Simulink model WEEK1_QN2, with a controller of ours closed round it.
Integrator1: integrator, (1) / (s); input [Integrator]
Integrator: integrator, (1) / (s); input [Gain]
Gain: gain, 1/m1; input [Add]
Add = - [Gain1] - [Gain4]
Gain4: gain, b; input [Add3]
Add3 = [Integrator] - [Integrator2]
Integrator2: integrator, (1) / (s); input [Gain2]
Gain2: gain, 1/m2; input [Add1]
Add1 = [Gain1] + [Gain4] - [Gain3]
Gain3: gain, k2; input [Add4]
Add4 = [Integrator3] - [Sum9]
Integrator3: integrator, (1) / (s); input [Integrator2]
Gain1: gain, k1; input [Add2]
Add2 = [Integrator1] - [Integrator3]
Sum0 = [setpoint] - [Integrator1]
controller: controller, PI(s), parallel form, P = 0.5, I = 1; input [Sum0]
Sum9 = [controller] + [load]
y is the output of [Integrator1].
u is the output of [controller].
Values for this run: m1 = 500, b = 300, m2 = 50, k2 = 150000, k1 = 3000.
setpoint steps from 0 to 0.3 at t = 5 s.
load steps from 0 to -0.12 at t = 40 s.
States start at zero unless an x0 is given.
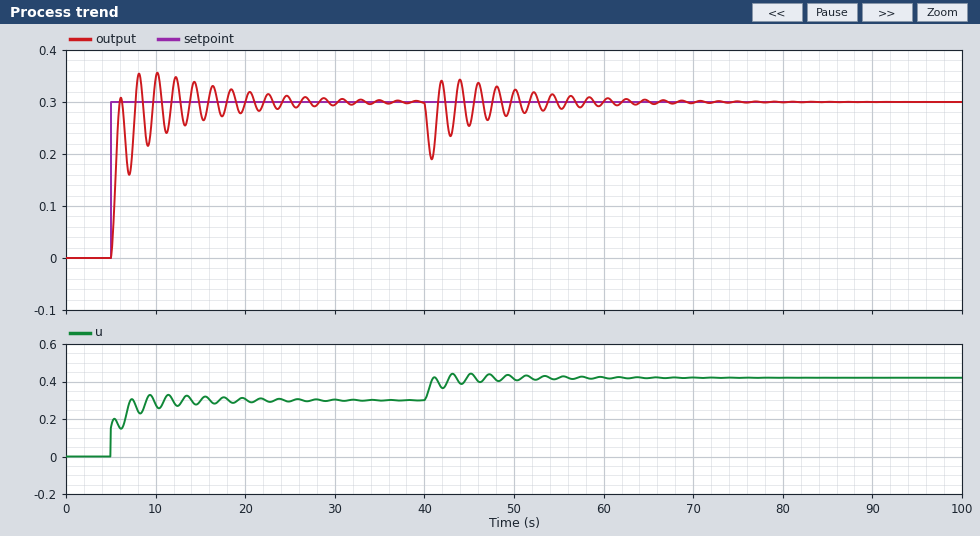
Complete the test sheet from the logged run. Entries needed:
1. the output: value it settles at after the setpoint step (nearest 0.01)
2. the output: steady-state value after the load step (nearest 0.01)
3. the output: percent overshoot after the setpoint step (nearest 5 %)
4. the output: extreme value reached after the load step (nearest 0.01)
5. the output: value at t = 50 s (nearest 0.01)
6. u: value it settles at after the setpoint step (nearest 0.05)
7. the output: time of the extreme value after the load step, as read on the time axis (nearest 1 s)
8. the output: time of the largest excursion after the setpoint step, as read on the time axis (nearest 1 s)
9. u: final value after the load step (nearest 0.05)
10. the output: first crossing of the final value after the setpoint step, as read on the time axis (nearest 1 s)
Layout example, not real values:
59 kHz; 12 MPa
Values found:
0.30; 0.30; 20 %; 0.19; 0.32; 0.30; 41 s; 10 s; 0.40; 6 s
